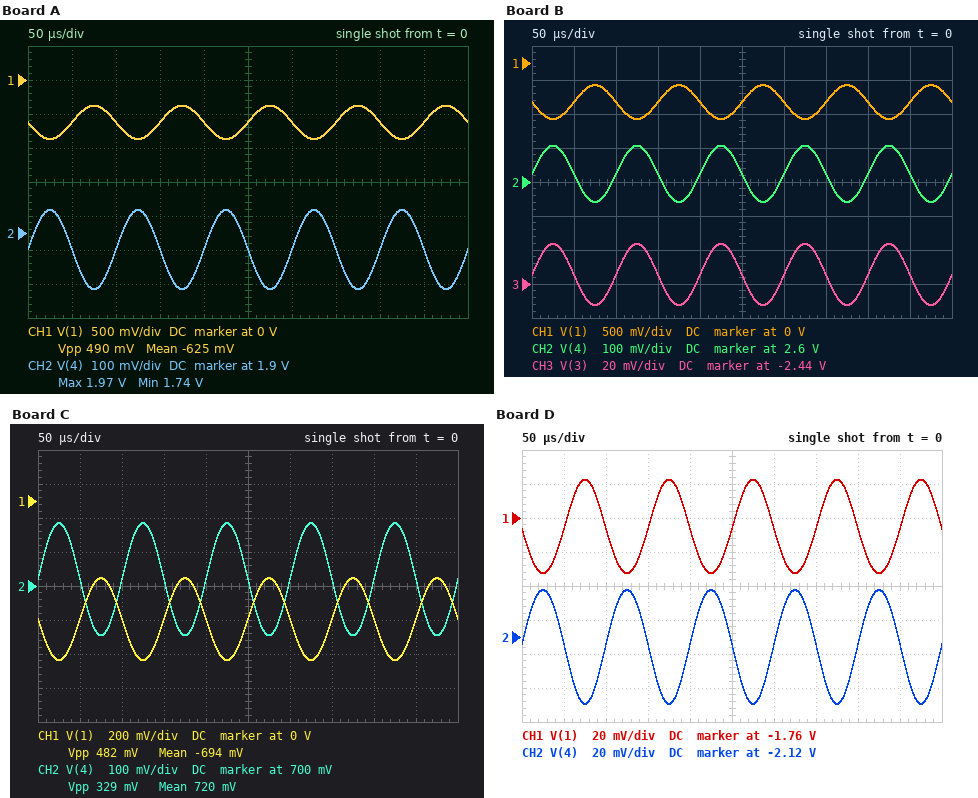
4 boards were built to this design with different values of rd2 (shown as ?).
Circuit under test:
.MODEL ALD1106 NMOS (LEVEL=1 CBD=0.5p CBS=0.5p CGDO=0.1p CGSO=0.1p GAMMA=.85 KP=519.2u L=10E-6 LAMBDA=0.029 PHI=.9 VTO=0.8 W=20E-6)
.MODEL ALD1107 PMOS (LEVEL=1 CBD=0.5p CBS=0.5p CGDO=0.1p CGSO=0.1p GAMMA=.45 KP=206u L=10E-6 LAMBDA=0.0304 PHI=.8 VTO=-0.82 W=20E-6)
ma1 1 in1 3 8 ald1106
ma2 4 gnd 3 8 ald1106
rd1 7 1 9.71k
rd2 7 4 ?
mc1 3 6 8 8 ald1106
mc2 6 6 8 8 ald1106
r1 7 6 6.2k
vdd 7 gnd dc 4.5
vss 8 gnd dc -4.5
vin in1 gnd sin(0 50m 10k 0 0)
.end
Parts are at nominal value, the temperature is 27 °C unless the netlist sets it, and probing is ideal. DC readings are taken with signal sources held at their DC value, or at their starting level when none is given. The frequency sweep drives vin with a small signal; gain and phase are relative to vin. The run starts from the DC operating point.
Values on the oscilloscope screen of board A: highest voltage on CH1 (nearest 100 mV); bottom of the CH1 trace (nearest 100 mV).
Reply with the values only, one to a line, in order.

-400 mV
-900 mV
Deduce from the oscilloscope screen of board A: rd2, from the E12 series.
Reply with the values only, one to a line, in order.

4.7 kΩ
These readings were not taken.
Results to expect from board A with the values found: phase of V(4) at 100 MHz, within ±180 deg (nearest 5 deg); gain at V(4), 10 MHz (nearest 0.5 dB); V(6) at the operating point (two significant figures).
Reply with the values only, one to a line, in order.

-35 deg
7.5 dB
-2.3 V
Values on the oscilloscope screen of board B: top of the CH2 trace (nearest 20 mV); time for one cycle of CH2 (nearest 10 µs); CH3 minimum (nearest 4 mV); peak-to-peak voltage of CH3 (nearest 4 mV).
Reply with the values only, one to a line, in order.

2.70 V
100 µs
-2.452 V
36 mV
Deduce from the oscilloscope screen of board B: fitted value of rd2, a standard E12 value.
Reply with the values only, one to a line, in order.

3.3 kΩ
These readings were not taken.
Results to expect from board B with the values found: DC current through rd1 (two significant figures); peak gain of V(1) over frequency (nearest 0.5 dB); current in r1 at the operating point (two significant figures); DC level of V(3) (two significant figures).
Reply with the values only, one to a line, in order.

520 µA
14.0 dB
1.1 mA
-2.4 V
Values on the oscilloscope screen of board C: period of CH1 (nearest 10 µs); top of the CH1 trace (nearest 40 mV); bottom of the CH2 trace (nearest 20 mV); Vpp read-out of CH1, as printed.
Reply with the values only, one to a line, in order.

100 µs
-440 mV
560 mV
482 mV
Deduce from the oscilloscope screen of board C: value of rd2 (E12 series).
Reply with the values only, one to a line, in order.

6.8 kΩ
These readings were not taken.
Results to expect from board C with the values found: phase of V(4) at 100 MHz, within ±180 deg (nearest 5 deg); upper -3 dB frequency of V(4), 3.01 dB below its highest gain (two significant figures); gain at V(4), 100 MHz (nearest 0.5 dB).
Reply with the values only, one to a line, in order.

-45 deg
140 MHz
8.5 dB
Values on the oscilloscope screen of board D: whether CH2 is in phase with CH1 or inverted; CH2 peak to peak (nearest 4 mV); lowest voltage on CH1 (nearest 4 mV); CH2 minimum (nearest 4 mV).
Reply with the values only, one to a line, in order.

inverted
68 mV
-1.792 V
-2.160 V
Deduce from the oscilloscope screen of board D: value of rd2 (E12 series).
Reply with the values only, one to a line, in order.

15 kΩ
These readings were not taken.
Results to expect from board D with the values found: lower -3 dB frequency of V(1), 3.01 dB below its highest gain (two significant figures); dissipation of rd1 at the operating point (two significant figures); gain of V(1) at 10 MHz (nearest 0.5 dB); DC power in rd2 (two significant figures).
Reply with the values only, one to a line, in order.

23 MHz
4.0 mW
-4.5 dB
2.9 mW
